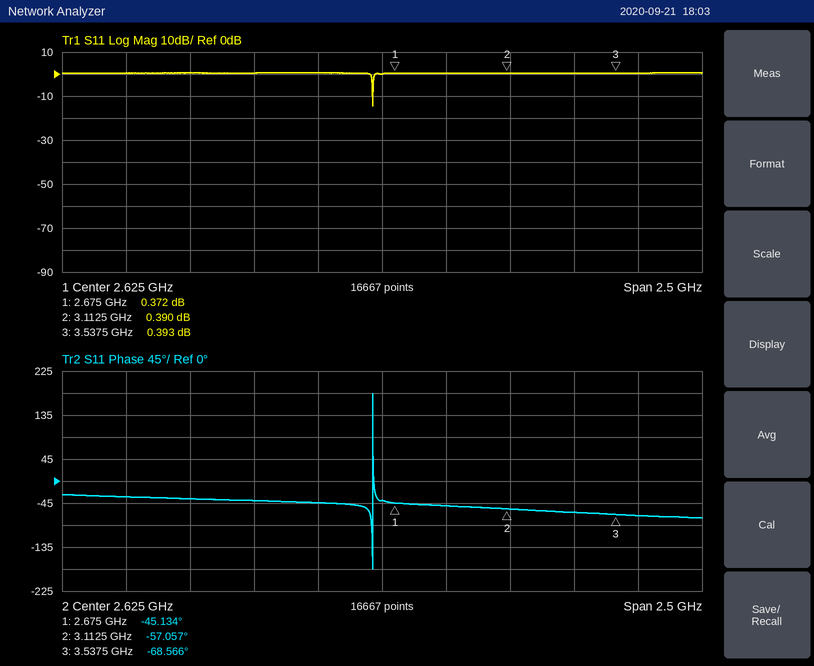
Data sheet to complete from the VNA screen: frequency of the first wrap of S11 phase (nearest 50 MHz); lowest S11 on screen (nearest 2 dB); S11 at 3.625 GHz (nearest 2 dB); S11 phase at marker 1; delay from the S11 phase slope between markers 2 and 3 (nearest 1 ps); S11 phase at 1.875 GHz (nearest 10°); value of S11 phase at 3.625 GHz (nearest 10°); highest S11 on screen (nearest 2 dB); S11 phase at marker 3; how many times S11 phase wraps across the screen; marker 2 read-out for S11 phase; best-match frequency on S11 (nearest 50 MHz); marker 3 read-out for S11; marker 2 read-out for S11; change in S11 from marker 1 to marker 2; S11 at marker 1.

2.60 GHz
-14 dB
0 dB
-45.134°
75 ps
-40°
-70°
0 dB
-68.566°
1
-57.057°
2.60 GHz
0.393 dB
0.390 dB
0.018 dB
0.372 dB
